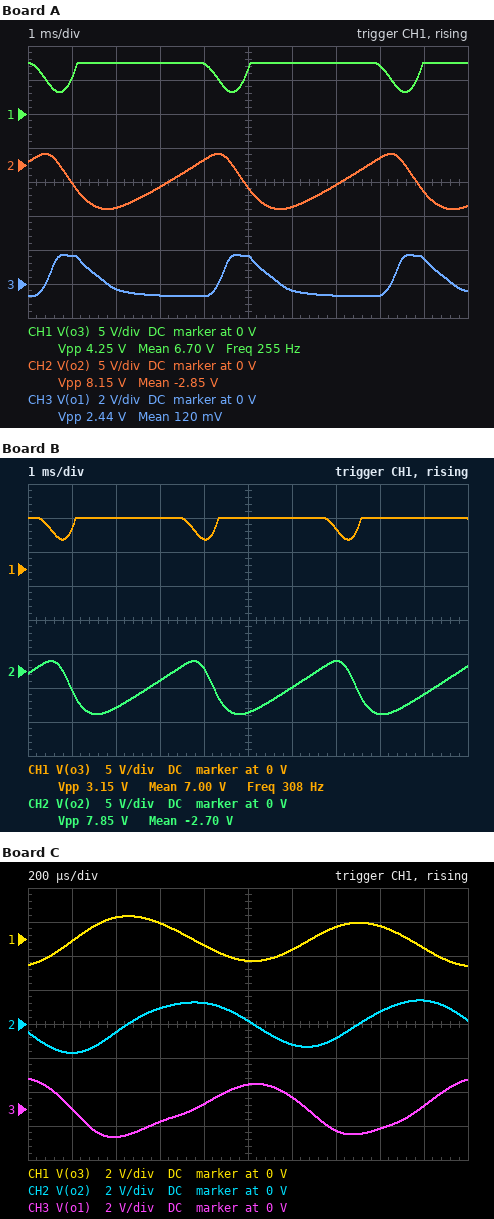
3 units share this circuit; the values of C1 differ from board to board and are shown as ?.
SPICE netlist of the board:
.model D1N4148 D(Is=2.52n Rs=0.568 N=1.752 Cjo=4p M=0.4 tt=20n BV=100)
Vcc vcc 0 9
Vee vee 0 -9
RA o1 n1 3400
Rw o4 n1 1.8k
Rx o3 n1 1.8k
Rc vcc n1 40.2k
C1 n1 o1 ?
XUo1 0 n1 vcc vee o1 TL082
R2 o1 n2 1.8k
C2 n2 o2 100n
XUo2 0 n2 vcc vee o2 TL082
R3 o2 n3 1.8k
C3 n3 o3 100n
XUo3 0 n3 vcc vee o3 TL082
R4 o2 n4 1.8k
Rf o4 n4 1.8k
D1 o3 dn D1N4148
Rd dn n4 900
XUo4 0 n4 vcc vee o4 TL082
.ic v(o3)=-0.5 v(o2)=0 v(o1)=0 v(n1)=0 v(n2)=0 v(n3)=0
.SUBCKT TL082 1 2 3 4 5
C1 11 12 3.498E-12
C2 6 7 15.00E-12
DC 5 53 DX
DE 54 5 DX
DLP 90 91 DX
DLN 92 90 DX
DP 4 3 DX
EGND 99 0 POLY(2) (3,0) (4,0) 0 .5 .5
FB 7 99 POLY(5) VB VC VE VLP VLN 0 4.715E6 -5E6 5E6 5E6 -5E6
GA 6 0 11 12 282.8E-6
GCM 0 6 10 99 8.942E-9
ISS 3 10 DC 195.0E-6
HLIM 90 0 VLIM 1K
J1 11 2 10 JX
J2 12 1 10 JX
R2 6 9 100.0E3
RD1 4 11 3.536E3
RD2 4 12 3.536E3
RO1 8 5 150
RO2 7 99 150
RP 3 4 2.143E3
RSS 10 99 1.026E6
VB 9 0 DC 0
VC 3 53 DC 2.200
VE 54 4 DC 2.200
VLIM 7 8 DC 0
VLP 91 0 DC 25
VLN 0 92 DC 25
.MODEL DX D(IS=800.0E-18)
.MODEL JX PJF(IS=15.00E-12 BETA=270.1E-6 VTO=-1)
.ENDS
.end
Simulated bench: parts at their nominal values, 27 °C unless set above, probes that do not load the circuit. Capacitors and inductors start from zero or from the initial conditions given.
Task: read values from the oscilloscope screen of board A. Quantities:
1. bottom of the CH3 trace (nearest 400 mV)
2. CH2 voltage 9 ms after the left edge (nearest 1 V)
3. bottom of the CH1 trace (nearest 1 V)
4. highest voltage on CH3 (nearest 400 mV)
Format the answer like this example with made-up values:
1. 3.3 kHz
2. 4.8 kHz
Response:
1. -800 mV
2. -4 V
3. 3 V
4. 1.6 V
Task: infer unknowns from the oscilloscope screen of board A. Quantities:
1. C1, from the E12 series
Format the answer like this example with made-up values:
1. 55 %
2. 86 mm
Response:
1. 220 nF
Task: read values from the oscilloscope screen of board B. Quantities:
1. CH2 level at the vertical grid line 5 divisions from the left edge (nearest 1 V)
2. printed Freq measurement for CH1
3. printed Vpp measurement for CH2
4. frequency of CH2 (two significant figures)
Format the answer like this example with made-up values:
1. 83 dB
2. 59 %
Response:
1. -6 V
2. 308 Hz
3. 7.85 V
4. 310 Hz
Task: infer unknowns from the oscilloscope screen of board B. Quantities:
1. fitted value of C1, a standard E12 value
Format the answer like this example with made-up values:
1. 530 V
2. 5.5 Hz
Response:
1. 120 nF
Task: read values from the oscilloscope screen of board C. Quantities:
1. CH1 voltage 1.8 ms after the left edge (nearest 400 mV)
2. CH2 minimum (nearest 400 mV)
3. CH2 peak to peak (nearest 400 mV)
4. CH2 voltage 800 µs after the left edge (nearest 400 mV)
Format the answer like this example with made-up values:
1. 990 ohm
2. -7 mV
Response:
1. -400 mV
2. -1.6 V
3. 3.2 V
4. 1.2 V
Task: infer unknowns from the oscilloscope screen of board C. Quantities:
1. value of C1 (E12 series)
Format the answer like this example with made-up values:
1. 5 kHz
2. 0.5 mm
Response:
1. 82 nF
